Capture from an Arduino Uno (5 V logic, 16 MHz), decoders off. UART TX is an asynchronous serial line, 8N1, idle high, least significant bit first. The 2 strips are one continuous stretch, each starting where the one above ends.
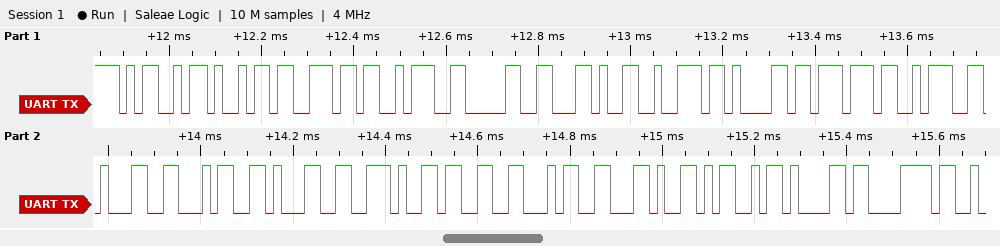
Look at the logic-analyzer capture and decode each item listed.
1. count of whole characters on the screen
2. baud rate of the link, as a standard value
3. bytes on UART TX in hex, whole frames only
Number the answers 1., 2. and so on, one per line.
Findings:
1. 20
2. 57600 baud
3. 4D 69 6E 3A 30 2C 72 61 77 3A 31 34 31 2E 33 34 2C 4D 61 78
